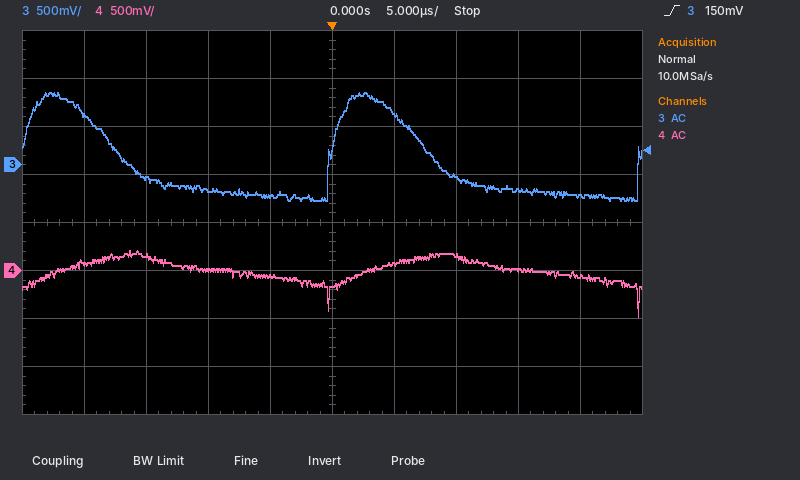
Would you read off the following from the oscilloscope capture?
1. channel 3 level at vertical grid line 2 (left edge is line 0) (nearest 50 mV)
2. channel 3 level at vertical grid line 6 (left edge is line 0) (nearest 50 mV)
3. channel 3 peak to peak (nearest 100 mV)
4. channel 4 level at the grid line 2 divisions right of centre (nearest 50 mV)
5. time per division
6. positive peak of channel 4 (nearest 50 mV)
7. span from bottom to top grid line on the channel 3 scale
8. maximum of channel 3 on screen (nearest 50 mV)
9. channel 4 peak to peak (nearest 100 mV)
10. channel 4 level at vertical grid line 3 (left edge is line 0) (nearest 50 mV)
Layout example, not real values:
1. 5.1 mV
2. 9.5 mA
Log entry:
1. -150 mV
2. 550 mV
3. 1.10 V
4. 150 mV
5. 5 µs
6. 200 mV
7. 4 V
8. 750 mV
9. 700 mV
10. 0 mV
